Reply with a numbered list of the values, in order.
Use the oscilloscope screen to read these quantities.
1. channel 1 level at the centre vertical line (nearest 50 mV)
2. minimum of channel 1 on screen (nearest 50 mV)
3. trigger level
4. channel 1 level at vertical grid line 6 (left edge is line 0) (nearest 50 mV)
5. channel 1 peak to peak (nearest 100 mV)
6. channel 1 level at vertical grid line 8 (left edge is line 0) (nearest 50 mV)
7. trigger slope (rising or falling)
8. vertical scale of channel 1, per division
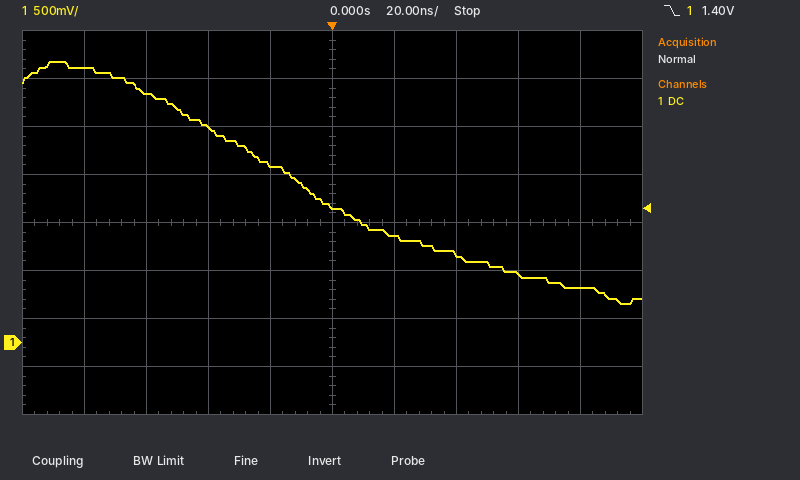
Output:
1. 1.40 V
2. 400 mV
3. 1.40 V
4. 1.10 V
5. 2.50 V
6. 700 mV
7. falling
8. 500 mV
